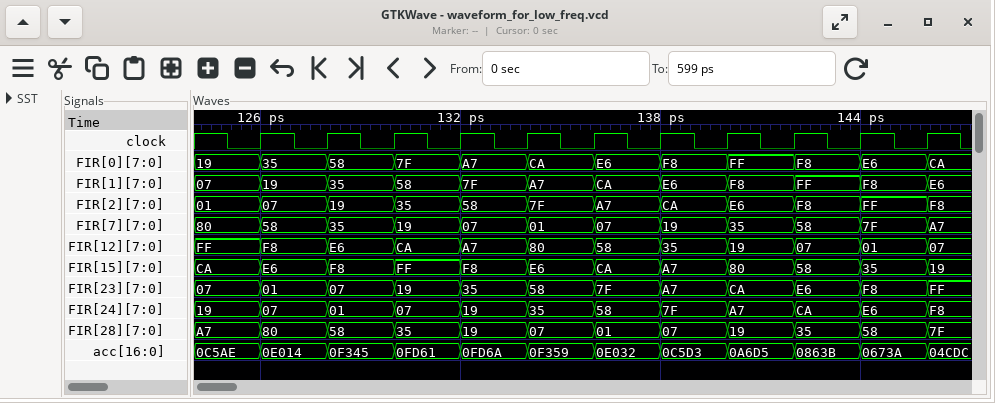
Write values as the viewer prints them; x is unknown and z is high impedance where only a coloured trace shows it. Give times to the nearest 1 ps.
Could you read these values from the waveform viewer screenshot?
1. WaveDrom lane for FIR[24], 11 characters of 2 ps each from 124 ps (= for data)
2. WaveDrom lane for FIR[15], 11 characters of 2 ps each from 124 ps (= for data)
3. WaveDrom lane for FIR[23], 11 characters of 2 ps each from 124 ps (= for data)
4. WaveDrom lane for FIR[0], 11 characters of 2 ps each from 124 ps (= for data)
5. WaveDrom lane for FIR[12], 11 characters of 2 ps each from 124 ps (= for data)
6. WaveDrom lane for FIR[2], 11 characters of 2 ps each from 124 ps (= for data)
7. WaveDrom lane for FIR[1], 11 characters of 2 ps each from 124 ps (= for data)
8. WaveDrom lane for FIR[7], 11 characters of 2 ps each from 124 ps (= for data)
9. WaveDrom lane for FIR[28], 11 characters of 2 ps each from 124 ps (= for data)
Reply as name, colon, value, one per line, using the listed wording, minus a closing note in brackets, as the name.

WaveDrom lane for FIR[24], 11 characters of 2 ps each from 124 ps: {name: 'FIR[24]', wave: '===========', data: '19 07 01 07 19 35 58 7F A7 CA E6'}
WaveDrom lane for FIR[15], 11 characters of 2 ps each from 124 ps: {name: 'FIR[15]', wave: '===========', data: 'CA E6 F8 FF F8 E6 CA A7 80 58 35'}
WaveDrom lane for FIR[23], 11 characters of 2 ps each from 124 ps: {name: 'FIR[23]', wave: '===========', data: '07 01 07 19 35 58 7F A7 CA E6 F8'}
WaveDrom lane for FIR[0], 11 characters of 2 ps each from 124 ps: {name: 'FIR[0]', wave: '===========', data: '19 35 58 7F A7 CA E6 F8 FF F8 E6'}
WaveDrom lane for FIR[12], 11 characters of 2 ps each from 124 ps: {name: 'FIR[12]', wave: '===========', data: 'FF F8 E6 CA A7 80 58 35 19 07 01'}
WaveDrom lane for FIR[2], 11 characters of 2 ps each from 124 ps: {name: 'FIR[2]', wave: '===========', data: '01 07 19 35 58 7F A7 CA E6 F8 FF'}
WaveDrom lane for FIR[1], 11 characters of 2 ps each from 124 ps: {name: 'FIR[1]', wave: '===========', data: '07 19 35 58 7F A7 CA E6 F8 FF F8'}
WaveDrom lane for FIR[7], 11 characters of 2 ps each from 124 ps: {name: 'FIR[7]', wave: '===========', data: '80 58 35 19 07 01 07 19 35 58 7F'}
WaveDrom lane for FIR[28], 11 characters of 2 ps each from 124 ps: {name: 'FIR[28]', wave: '===========', data: 'A7 80 58 35 19 07 01 07 19 35 58'}
